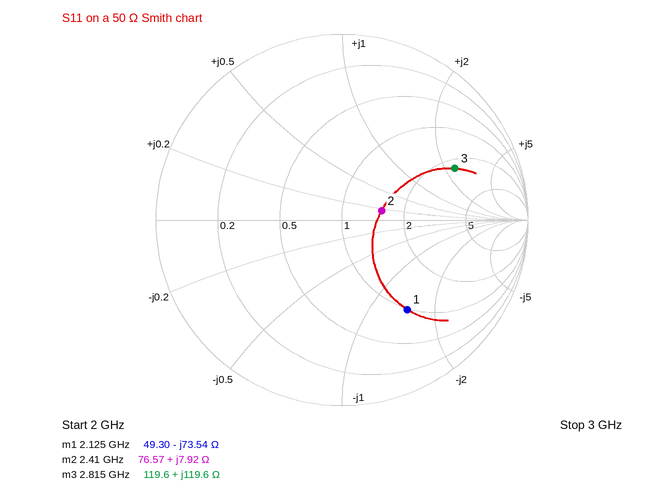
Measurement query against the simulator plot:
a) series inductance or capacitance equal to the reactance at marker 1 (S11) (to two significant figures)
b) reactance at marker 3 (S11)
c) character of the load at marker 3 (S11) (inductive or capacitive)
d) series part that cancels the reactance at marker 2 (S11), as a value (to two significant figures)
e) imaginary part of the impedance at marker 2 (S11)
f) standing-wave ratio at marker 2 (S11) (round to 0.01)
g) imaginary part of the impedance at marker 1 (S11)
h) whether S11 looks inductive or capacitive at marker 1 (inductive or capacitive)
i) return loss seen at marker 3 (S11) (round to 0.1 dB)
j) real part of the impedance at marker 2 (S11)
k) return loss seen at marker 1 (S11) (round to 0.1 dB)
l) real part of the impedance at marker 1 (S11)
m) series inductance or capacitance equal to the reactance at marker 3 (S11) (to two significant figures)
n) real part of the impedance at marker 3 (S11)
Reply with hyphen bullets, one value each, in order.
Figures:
- 1.0 pF
- +119.6 Ω
- inductive
- 8.3 pF
- +7.92 Ω
- 1.56
- -73.54 Ω
- capacitive
- 3.5 dB
- 76.57 Ω
- 4.5 dB
- 49.30 Ω
- 6.8 nH
- 119.6 Ω
